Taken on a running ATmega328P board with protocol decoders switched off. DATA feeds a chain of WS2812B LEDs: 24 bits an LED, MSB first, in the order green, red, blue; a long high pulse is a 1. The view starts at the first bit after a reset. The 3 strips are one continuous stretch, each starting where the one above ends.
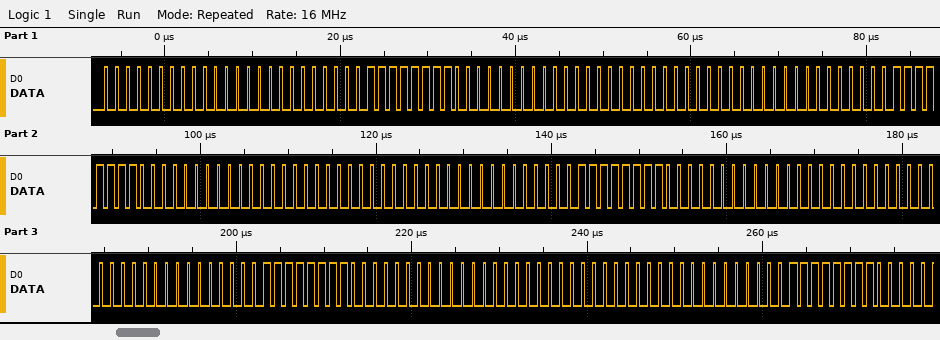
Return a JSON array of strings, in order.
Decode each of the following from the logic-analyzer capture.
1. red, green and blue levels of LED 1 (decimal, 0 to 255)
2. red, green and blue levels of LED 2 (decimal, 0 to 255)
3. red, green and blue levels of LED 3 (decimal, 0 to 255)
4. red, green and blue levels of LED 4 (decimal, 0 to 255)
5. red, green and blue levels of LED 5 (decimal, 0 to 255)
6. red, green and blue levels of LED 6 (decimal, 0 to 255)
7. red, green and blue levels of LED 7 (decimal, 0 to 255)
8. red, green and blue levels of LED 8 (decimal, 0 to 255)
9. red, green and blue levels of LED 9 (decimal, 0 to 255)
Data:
["0, 0, 0", "0, 255, 0", "0, 0, 0", "0, 255, 0", "0, 0, 0", "0, 255, 0", "0, 0, 0", "0, 255, 0", "0, 0, 0"]
